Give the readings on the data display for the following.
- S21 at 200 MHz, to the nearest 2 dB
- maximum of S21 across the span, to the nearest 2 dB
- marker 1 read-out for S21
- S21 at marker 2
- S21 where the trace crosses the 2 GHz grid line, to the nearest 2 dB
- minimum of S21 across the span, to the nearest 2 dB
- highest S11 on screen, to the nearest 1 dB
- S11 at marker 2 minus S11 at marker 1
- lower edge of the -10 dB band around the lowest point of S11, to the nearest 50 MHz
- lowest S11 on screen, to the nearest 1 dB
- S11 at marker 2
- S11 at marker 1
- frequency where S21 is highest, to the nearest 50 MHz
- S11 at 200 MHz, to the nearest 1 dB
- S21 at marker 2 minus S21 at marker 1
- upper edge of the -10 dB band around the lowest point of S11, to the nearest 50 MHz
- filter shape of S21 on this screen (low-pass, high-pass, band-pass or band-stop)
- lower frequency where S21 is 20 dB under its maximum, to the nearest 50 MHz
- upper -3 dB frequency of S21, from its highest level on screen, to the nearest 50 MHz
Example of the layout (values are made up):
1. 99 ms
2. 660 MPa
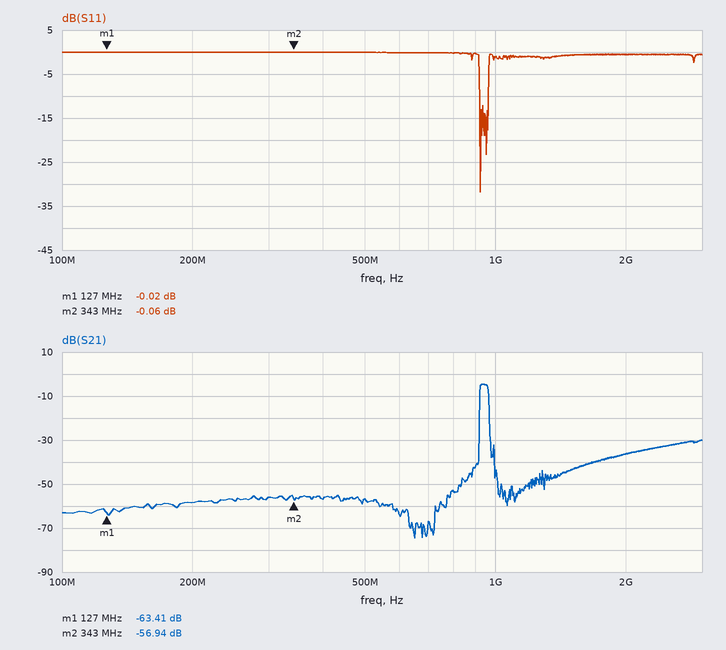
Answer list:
1. -58 dB
2. -4 dB
3. -63.41 dB
4. -56.94 dB
5. -36 dB
6. -74 dB
7. 0 dB
8. -0.04 dB
9. 900 MHz
10. -32 dB
11. -0.06 dB
12. -0.02 dB
13. 950 MHz
14. 0 dB
15. 6.47 dB
16. 950 MHz
17. band-pass
18. 900 MHz
19. 950 MHz
